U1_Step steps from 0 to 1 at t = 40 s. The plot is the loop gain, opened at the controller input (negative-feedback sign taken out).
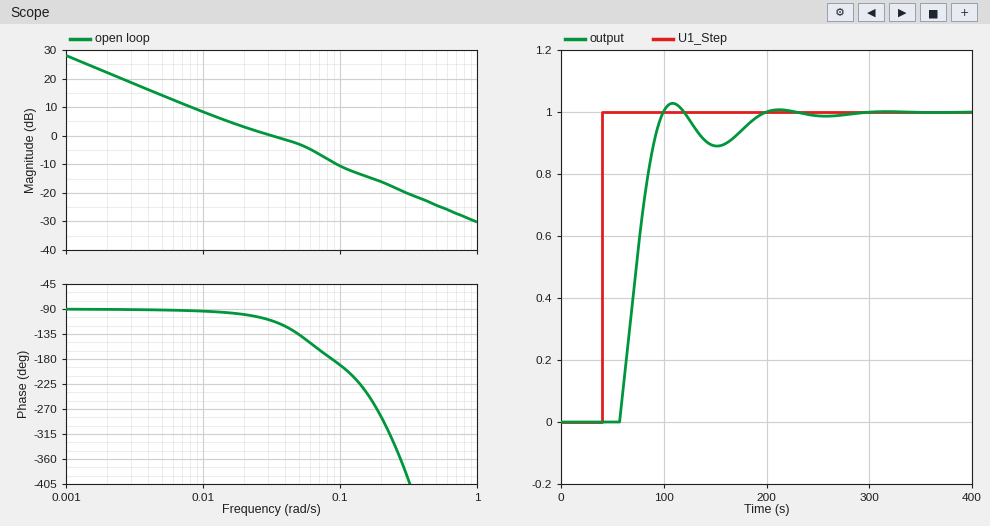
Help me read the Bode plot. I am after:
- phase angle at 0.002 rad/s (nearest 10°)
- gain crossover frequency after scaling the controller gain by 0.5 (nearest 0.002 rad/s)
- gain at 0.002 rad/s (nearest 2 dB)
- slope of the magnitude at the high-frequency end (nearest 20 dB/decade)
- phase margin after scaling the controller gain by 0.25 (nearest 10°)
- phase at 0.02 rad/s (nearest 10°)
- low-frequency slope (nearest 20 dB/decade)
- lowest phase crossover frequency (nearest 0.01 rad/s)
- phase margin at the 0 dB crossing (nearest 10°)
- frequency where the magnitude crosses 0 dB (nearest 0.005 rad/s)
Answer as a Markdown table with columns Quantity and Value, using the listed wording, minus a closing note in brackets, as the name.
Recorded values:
| Quantity | Value |
|---|---|
| phase angle at 0.002 rad/s | -90° |
| gain crossover frequency after scaling the controller gain by 0.5 | 0.014 rad/s |
| gain at 0.002 rad/s | 22 dB |
| slope of the magnitude at the high-frequency end | -20 dB/decade |
| phase margin after scaling the controller gain by 0.25 | 90° |
| phase at 0.02 rad/s | -100° |
| low-frequency slope | -20 dB/decade |
| lowest phase crossover frequency | 0.09 rad/s |
| phase margin at the 0 dB crossing | 70° |
| frequency where the magnitude crosses 0 dB | 0.030 rad/s |
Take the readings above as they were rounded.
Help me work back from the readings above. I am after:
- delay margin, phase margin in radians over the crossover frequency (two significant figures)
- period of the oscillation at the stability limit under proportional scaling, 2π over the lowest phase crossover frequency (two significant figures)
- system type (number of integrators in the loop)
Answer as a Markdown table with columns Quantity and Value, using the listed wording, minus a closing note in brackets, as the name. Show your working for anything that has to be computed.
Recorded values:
| Quantity | Value |
|---|---|
| delay margin, phase margin in radians over the crossover frequency | 70 × π / 180 / 0.03 = 41 s |
| period of the oscillation at the stability limit under proportional scaling, 2π over the lowest phase crossover frequency | 2π / 0.09 = 70 s |
| system type | 1 |
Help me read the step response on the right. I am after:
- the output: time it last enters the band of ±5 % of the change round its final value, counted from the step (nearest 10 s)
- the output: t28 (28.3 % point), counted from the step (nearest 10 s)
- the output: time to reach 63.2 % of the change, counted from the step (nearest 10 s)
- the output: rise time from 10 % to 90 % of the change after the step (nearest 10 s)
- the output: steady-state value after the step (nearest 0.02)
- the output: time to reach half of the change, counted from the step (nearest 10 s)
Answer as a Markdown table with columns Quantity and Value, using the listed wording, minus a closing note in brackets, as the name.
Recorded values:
| Quantity | Value |
|---|---|
| the output: time it last enters the band of ±5 % of the change round its final value, counted from the step | 140 s |
| the output: t28 (28.3 % point), counted from the step | 30 s |
| the output: time to reach 63.2 % of the change, counted from the step | 40 s |
| the output: rise time from 10 % to 90 % of the change after the step | 30 s |
| the output: steady-state value after the step | 1.00 |
| the output: time to reach half of the change, counted from the step | 30 s |
